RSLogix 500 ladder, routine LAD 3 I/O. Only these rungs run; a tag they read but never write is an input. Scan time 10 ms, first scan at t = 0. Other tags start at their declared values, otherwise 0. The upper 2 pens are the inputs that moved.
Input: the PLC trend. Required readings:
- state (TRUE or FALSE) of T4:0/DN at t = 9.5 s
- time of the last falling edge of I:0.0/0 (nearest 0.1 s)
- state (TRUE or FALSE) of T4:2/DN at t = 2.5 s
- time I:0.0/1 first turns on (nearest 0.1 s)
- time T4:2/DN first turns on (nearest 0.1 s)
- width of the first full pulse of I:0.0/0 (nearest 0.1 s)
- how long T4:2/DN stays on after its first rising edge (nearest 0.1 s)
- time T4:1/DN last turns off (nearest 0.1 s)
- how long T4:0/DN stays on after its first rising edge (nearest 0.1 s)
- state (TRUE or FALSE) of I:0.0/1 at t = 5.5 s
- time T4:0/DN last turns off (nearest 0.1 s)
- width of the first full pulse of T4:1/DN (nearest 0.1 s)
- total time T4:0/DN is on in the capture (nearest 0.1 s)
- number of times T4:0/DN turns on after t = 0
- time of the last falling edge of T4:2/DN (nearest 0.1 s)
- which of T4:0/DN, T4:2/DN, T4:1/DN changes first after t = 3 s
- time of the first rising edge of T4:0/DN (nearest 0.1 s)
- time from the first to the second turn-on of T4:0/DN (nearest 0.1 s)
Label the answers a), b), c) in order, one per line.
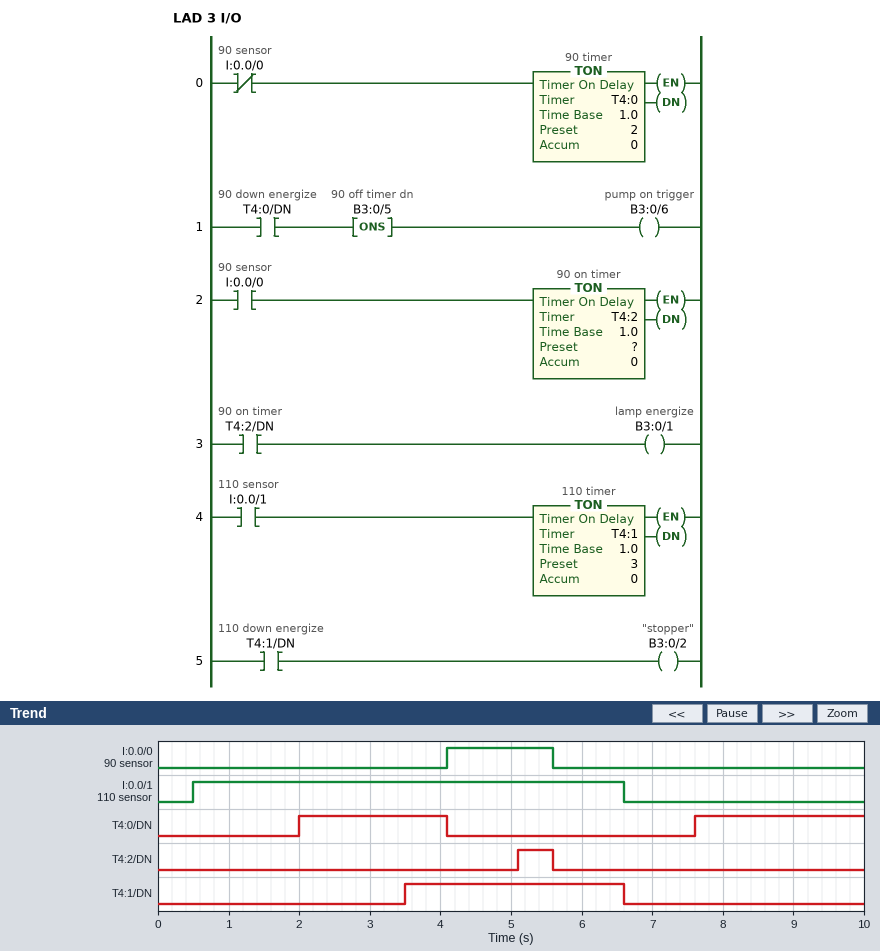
a) TRUE
b) 5.6 s
c) FALSE
d) 0.5 s
e) 5.1 s
f) 1.5 s
g) 0.5 s
h) 6.6 s
i) 2.1 s
j) TRUE
k) 4.1 s
l) 3.1 s
m) 4.5 s
n) 2
o) 5.6 s
p) T4:1/DN
q) 2.0 s
r) 5.6 s
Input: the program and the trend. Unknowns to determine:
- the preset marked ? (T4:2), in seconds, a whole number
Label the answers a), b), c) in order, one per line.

a) 1 s
